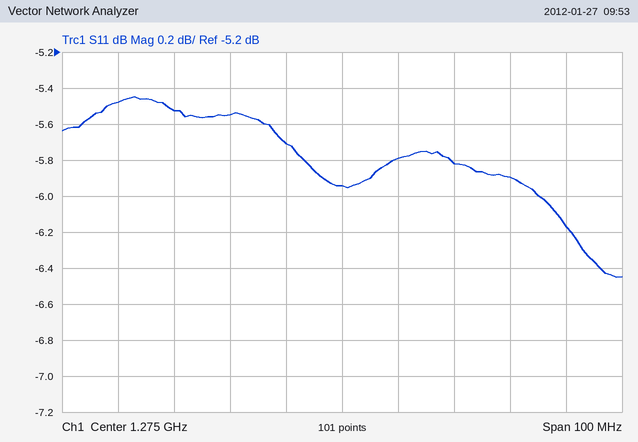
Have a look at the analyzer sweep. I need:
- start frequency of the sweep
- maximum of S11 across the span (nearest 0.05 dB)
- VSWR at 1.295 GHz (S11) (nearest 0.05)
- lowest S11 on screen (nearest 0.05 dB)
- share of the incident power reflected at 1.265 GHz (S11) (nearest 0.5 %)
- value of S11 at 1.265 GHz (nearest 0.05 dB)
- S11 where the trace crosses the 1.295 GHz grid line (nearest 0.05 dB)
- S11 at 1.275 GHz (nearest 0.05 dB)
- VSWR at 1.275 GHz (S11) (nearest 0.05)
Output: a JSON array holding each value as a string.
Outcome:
["1.225 GHz", "-5.45 dB", "3.10", "-6.45 dB", "27.0 %", "-5.70 dB", "-5.80 dB", "-5.95 dB", "3.05"]
